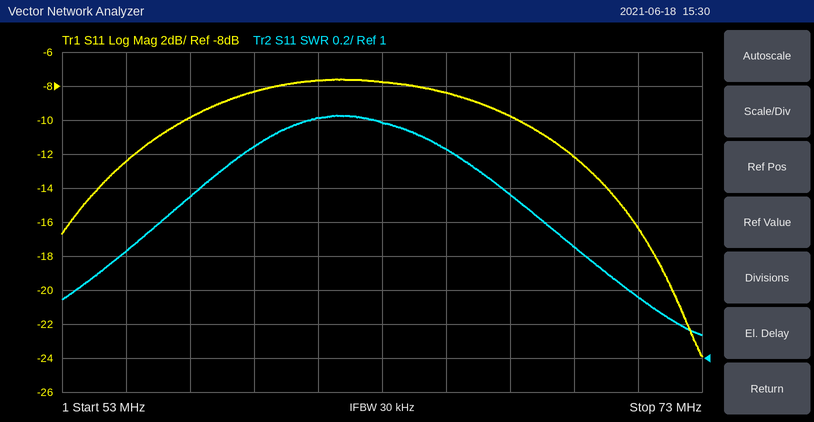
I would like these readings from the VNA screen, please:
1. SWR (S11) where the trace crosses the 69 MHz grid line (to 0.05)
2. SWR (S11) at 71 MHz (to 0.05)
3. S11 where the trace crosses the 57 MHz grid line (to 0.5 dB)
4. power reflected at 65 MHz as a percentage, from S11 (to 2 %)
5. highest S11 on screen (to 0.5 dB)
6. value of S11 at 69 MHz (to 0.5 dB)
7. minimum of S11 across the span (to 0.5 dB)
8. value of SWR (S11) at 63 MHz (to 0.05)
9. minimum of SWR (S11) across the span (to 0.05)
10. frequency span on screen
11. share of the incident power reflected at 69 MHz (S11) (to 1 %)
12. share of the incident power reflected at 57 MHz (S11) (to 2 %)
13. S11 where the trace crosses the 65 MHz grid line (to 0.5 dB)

1.65
1.35
-10.0 dB
14 %
-7.5 dB
-12.0 dB
-24.0 dB
2.40
1.15
20 MHz
6 %
10 %
-8.5 dB
